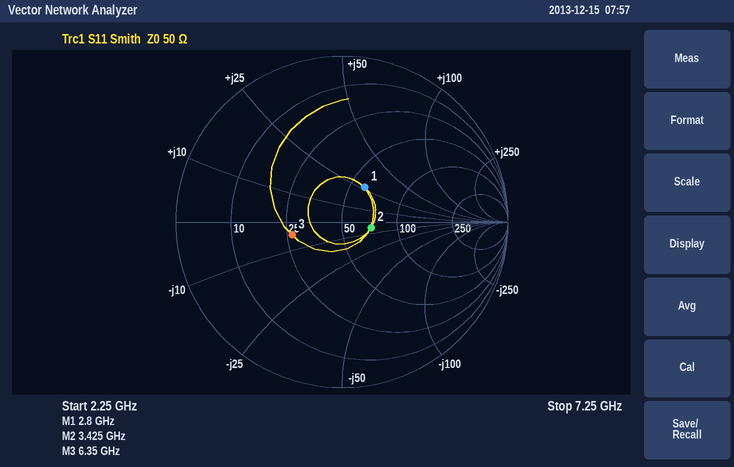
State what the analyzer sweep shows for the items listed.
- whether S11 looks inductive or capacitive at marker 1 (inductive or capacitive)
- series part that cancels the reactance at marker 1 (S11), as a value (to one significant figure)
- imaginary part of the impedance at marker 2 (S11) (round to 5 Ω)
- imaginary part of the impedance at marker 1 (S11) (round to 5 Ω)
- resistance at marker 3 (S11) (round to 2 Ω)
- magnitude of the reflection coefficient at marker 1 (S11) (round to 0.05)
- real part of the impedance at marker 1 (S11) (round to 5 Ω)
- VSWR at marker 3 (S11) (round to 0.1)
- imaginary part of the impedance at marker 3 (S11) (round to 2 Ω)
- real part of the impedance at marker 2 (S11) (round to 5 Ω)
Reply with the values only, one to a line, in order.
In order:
inductive
2 pF
-5 Ω
+25 Ω
26 Ω
0.25
60 Ω
1.9
-4 Ω
70 Ω
